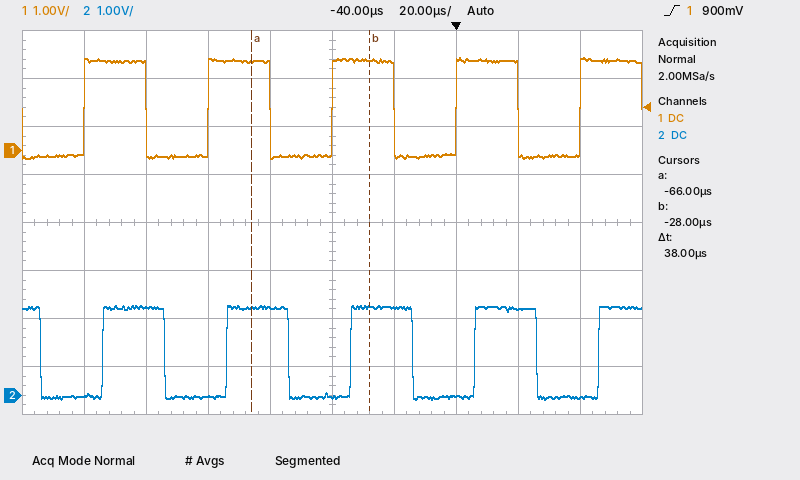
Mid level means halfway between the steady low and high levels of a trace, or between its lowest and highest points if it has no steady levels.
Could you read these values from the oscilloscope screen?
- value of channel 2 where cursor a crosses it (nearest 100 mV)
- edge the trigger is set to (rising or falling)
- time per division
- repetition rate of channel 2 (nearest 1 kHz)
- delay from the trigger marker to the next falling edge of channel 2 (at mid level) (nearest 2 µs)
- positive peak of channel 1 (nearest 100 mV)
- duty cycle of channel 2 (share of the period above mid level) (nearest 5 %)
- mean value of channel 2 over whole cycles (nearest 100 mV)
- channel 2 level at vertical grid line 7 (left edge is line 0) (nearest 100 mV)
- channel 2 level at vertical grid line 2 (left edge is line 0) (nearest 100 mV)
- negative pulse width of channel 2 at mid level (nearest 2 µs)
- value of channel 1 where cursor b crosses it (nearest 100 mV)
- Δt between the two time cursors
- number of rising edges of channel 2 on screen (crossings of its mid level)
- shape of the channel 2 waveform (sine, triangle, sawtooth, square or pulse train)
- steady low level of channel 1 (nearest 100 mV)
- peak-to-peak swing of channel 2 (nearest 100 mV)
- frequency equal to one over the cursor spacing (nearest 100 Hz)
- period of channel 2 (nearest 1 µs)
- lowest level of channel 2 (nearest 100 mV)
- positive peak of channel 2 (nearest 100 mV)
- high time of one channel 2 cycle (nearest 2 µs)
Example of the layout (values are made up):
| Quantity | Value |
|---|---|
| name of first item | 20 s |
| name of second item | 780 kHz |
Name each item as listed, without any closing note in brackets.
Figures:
| Quantity | Value |
|---|---|
| value of channel 2 where cursor a crosses it | 1.8 V |
| edge the trigger is set to | rising |
| time per division | 20 µs |
| repetition rate of channel 2 | 25 kHz |
| delay from the trigger marker to the next falling edge of channel 2 (at mid level) | 26 µs |
| positive peak of channel 1 | 1.9 V |
| duty cycle of channel 2 (share of the period above mid level) | 50 % |
| mean value of channel 2 over whole cycles | 900 mV |
| channel 2 level at vertical grid line 7 (left edge is line 0) | 0.0 V |
| channel 2 level at vertical grid line 2 (left edge is line 0) | 1.8 V |
| negative pulse width of channel 2 at mid level | 20 µs |
| value of channel 1 where cursor b crosses it | 1.9 V |
| Δt between the two time cursors | 38 µs |
| number of rising edges of channel 2 on screen | 5 |
| shape of the channel 2 waveform | square |
| steady low level of channel 1 | -100 mV |
| peak-to-peak swing of channel 2 | 2.0 V |
| frequency equal to one over the cursor spacing | 26.3 kHz |
| period of channel 2 | 40 µs |
| lowest level of channel 2 | -100 mV |
| positive peak of channel 2 | 1.9 V |
| high time of one channel 2 cycle | 20 µs |
